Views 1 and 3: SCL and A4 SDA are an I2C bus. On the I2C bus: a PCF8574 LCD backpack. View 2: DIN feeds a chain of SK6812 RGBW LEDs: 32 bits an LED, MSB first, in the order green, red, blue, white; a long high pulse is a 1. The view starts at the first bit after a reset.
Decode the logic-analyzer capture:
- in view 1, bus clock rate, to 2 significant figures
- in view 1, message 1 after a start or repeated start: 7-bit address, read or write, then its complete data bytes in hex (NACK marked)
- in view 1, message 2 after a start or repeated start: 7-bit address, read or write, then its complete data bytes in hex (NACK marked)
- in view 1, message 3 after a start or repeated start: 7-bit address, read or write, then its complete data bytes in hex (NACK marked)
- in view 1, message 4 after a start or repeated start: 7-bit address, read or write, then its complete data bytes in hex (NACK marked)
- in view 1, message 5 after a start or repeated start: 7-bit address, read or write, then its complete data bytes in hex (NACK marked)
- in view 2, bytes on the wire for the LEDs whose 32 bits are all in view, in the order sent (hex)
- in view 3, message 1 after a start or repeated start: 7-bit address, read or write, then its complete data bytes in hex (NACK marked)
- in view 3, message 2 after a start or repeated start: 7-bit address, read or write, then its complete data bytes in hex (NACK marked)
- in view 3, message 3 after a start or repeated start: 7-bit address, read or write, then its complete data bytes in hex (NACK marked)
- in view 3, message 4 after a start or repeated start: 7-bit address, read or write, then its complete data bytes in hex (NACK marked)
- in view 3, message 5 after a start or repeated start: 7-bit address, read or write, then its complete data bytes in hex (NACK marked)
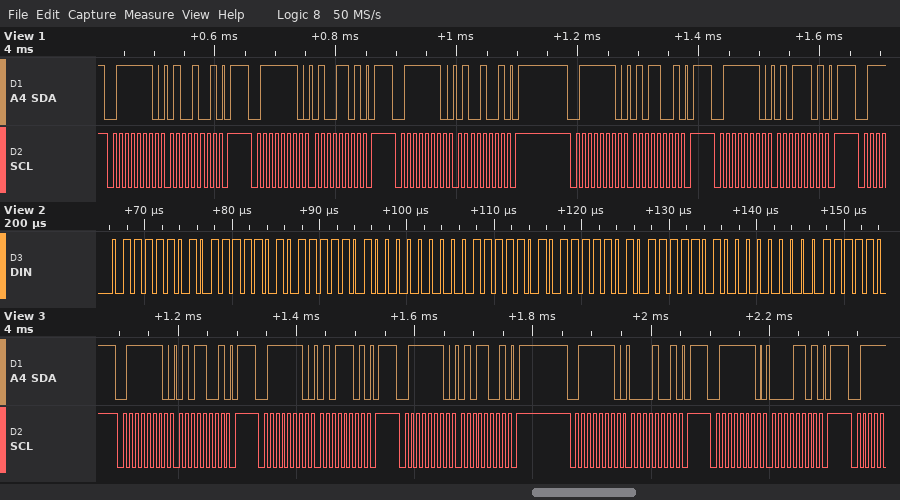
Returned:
100 kHz
0x3F write: 49
0x3F write: 4D
0x3F write: 49
0x3F write: 59
0x3F write: 5D
7D 7D 7D 00 7D 7D 7D 00
0x3F write: 59
0x3F write: 5D
0x3F write: 59
0x3F write: 09
0x3F write: 0D
